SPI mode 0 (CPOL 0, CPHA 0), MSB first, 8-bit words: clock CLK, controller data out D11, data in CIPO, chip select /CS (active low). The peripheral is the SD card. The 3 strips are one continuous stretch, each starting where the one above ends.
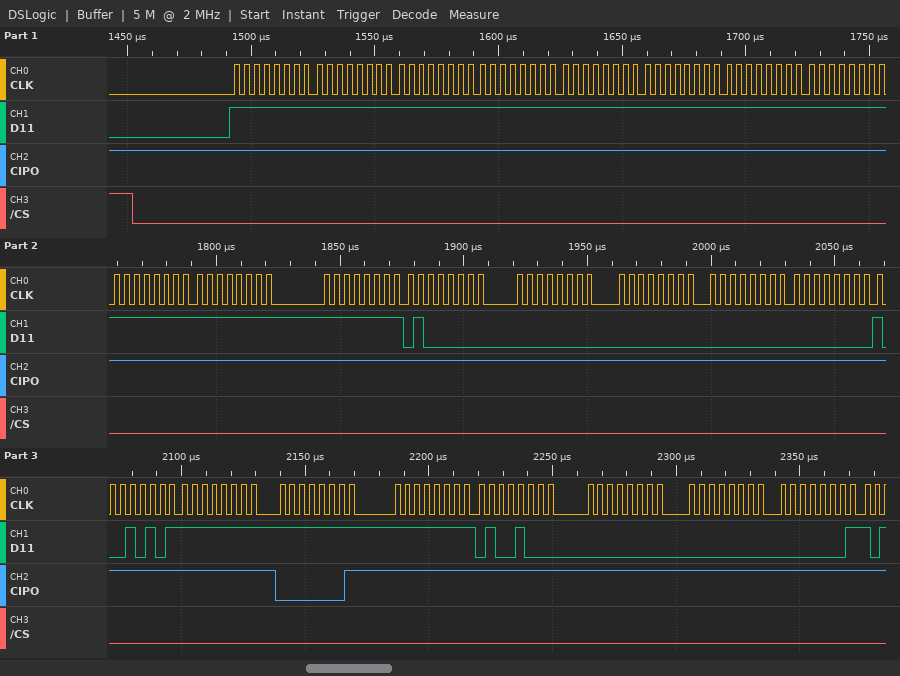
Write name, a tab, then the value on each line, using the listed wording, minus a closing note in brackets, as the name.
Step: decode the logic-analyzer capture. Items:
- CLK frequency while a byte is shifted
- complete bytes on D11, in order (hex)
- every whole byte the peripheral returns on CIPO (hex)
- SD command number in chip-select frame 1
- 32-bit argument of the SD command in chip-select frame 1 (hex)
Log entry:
CLK frequency while a byte is shifted	250 kHz
complete bytes on D11, in order	FF FF FF FF FF FF FF FF FF FF FF 40 00 00 00 00 95 FF FF FF 48 00 00 01
every whole byte the peripheral returns on CIPO	FF FF FF FF FF FF FF FF FF FF FF FF FF FF FF FF FF FF 01 FF FF FF FF FF
SD command number in chip-select frame 1	CMD0
32-bit argument of the SD command in chip-select frame 1	0x00000000
